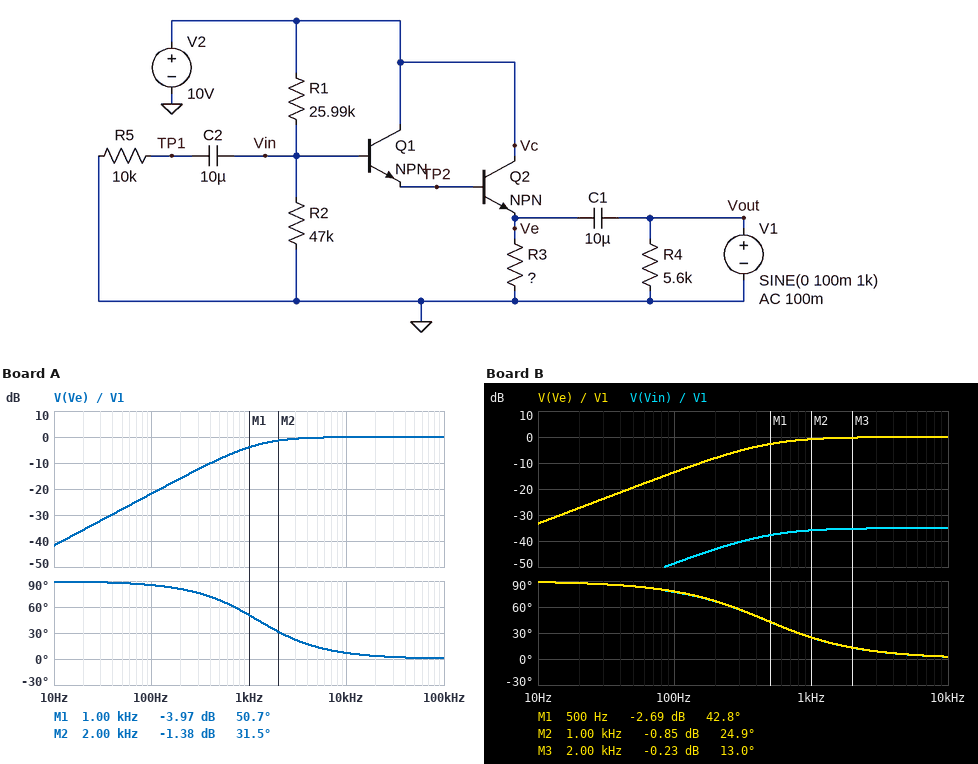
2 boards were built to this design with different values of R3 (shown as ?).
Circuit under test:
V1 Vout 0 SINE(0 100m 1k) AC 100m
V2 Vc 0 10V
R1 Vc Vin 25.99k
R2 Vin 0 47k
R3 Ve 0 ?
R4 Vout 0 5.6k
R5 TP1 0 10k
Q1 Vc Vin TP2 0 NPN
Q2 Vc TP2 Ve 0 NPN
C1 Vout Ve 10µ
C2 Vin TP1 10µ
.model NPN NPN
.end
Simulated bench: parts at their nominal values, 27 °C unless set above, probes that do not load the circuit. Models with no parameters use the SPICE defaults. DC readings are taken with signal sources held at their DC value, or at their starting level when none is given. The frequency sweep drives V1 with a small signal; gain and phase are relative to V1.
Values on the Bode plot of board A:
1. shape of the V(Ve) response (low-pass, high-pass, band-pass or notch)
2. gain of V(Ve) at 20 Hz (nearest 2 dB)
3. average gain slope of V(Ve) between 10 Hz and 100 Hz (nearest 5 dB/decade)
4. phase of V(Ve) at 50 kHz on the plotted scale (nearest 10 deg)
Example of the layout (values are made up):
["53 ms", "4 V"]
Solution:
["high-pass", "-36 dB", "20 dB/decade", "0 deg"]
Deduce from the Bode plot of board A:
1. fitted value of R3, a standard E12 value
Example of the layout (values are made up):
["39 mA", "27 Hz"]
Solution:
["1.2 kΩ"]
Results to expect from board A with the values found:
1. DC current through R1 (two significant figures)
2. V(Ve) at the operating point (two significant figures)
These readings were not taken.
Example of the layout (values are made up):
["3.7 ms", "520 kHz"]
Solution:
["140 µA", "4.9 V"]
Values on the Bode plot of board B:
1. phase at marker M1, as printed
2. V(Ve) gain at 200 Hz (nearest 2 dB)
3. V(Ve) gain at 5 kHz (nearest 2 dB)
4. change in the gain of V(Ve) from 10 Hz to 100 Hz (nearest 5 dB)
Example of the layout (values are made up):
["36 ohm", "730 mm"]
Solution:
["42.8 deg", "-8 dB", "0 dB", "20 dB"]
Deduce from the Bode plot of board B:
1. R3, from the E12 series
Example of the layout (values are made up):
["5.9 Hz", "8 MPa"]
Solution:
["3.3 kΩ"]
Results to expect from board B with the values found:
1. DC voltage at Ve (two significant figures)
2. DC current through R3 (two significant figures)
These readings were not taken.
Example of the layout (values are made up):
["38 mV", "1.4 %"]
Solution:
["5.0 V", "1.5 mA"]
